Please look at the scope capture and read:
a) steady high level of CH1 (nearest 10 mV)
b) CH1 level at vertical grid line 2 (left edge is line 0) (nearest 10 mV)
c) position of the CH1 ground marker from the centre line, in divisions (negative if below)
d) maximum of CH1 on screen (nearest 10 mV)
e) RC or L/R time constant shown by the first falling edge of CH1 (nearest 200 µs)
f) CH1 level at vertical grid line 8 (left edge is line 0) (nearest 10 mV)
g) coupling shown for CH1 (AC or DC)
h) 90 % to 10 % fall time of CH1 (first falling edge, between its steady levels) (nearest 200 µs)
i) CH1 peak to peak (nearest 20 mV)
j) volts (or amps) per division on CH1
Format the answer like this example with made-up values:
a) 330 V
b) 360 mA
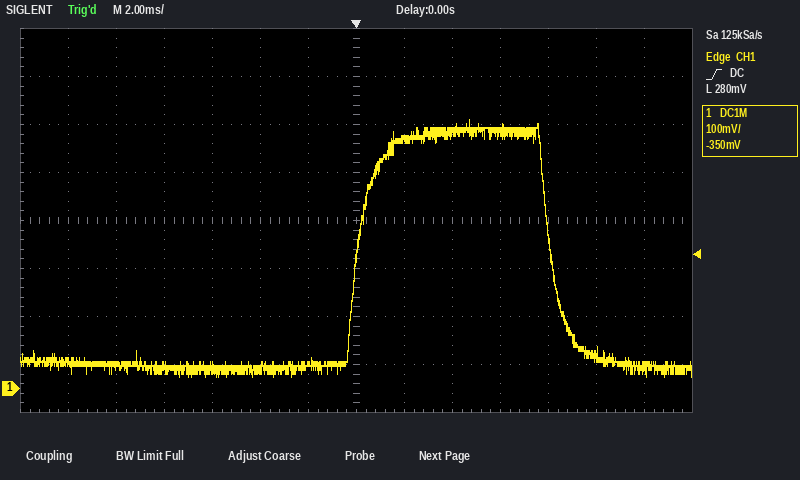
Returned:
a) 540 mV
b) 50 mV
c) -3.5 div
d) 560 mV
e) 600 µs
f) 520 mV
g) DC
h) 1.4 ms
i) 540 mV
j) 100 mV
